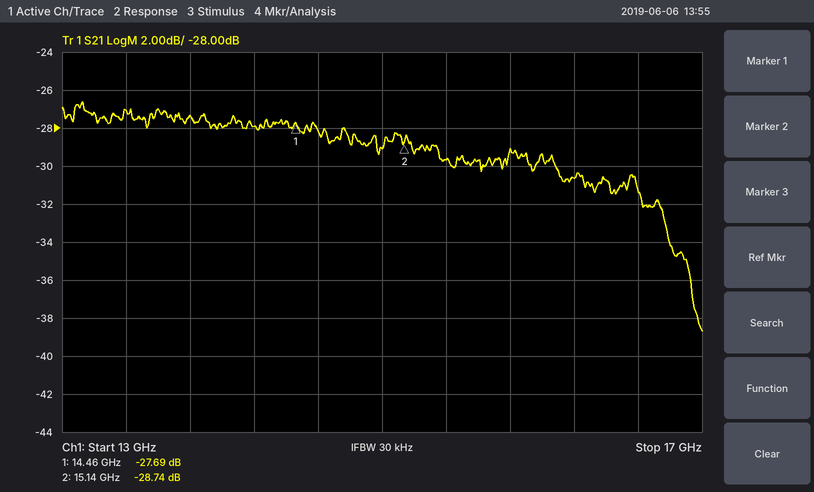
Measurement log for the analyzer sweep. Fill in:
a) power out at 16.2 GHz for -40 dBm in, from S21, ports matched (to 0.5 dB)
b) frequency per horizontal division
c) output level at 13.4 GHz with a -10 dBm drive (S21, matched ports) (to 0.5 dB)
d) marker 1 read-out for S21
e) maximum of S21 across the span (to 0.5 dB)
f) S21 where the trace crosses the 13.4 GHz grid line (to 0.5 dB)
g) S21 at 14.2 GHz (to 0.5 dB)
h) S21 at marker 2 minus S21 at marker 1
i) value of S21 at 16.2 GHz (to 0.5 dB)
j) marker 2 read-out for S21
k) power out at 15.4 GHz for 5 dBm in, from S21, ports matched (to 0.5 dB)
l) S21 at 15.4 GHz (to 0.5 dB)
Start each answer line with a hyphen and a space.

- -70.5 dBm
- 400 MHz
- -37.0 dBm
- -27.69 dB
- -26.5 dB
- -27.0 dB
- -28.0 dB
- -1.05 dB
- -30.5 dB
- -28.74 dB
- -24.5 dBm
- -29.5 dB
